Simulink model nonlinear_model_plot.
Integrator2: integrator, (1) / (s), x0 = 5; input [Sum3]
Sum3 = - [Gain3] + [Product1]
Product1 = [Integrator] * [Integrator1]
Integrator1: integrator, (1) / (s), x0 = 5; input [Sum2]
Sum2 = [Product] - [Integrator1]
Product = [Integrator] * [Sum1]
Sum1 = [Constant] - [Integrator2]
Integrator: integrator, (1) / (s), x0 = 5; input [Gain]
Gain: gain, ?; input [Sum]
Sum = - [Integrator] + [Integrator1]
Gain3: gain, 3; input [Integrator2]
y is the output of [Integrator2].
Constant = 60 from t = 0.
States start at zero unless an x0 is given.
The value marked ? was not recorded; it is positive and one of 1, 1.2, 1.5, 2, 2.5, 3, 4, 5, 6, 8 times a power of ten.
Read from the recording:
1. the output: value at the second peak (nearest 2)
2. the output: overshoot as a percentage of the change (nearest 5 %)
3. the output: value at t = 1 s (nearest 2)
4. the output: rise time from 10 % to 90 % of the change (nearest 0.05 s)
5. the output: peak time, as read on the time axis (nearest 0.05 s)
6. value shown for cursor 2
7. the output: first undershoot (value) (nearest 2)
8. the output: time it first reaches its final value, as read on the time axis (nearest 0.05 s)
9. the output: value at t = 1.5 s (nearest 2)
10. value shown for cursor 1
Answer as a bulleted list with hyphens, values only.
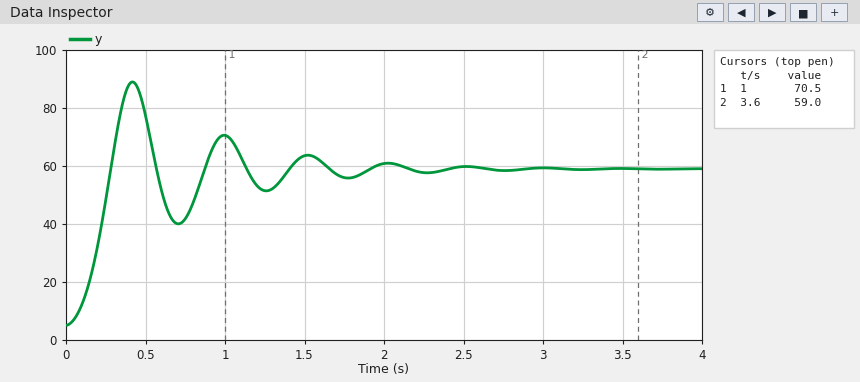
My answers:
- 70
- 55 %
- 70
- 0.20 s
- 0.40 s
- 59.0
- 40
- 0.30 s
- 64
- 70.5
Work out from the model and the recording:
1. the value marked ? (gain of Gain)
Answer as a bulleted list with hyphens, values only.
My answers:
- 0.5
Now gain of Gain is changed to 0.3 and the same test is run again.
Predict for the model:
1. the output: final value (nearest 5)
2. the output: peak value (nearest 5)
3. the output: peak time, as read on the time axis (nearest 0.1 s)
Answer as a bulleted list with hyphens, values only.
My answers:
- 60
- 85
- 0.5 s
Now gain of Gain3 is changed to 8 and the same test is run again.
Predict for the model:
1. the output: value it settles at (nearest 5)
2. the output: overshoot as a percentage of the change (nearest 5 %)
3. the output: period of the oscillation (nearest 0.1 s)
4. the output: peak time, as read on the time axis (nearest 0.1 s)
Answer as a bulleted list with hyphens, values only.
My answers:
- 60
- 35 %
- 0.4 s
- 0.4 s
